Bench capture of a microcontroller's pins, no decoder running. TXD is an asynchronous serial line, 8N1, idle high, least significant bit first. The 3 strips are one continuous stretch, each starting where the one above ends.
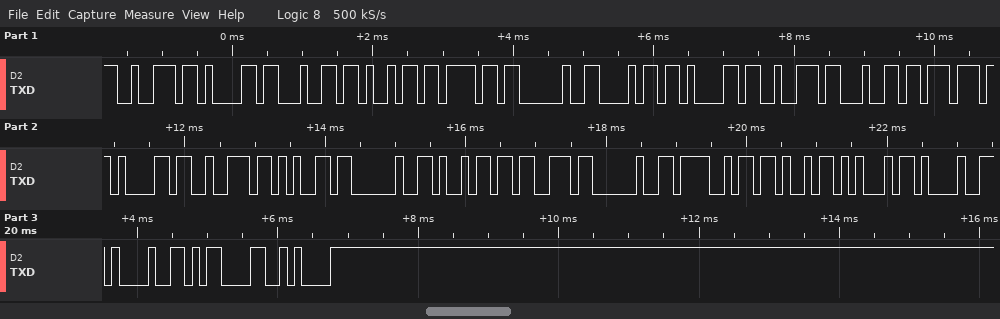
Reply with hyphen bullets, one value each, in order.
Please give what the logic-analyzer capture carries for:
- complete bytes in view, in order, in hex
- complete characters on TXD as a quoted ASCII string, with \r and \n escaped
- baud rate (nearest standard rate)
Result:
- 72 61 64 69 6F 20 68 61 72 64 77 61 72 65 20 69 73 20 4F 4B 45 21 21 0D 0A
- "radio hardware is OKE!!\r\n"
- 9600 baud
